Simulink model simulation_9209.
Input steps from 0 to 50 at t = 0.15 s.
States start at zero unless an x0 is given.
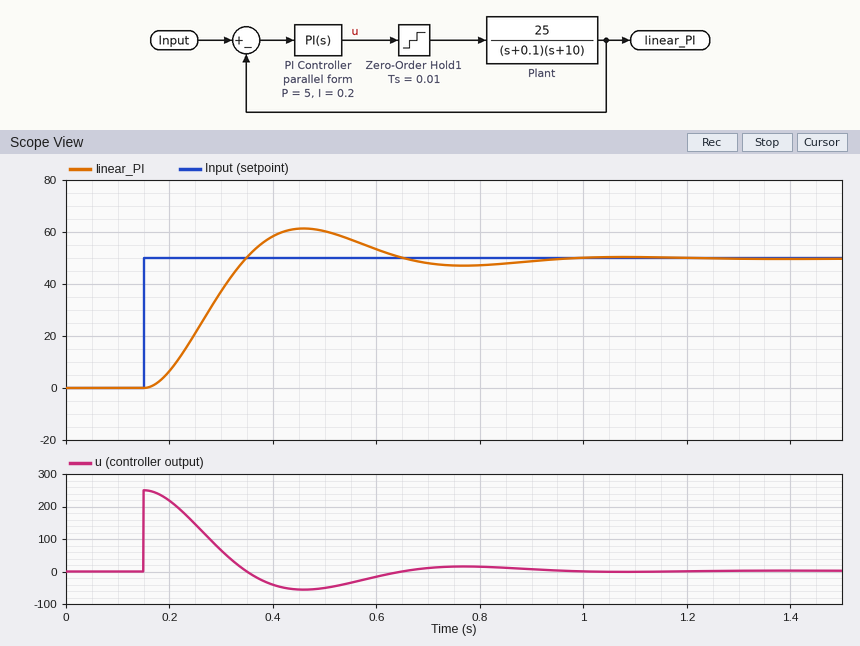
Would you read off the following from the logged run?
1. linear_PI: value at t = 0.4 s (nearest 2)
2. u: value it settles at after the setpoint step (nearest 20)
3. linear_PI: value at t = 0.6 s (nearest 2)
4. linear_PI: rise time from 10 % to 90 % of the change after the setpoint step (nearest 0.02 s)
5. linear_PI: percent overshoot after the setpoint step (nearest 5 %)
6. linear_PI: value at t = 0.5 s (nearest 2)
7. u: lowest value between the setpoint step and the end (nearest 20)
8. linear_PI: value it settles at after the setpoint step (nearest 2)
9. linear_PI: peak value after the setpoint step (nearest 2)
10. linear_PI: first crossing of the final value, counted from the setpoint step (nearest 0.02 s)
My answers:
58
0
54
0.14 s
25 %
60
-60
50
62
0.20 s
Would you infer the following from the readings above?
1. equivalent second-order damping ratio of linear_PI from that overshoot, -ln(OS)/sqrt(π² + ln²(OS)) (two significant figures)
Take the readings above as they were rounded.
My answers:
0.40
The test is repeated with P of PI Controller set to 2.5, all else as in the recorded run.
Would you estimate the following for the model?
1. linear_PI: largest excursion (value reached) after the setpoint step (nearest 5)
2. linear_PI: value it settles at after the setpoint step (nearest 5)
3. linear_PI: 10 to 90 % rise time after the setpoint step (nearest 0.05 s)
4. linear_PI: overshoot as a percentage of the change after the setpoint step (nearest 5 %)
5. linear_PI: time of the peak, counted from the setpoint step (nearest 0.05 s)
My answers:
55
50
0.25 s
10 %
0.50 s
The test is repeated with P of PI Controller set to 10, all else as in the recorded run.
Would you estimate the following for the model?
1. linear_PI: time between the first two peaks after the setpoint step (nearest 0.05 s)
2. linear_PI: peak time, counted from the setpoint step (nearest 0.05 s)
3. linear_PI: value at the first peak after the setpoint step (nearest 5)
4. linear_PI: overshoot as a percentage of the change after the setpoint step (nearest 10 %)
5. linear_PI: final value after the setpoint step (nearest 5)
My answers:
0.40 s
0.20 s
70
40 %
50
